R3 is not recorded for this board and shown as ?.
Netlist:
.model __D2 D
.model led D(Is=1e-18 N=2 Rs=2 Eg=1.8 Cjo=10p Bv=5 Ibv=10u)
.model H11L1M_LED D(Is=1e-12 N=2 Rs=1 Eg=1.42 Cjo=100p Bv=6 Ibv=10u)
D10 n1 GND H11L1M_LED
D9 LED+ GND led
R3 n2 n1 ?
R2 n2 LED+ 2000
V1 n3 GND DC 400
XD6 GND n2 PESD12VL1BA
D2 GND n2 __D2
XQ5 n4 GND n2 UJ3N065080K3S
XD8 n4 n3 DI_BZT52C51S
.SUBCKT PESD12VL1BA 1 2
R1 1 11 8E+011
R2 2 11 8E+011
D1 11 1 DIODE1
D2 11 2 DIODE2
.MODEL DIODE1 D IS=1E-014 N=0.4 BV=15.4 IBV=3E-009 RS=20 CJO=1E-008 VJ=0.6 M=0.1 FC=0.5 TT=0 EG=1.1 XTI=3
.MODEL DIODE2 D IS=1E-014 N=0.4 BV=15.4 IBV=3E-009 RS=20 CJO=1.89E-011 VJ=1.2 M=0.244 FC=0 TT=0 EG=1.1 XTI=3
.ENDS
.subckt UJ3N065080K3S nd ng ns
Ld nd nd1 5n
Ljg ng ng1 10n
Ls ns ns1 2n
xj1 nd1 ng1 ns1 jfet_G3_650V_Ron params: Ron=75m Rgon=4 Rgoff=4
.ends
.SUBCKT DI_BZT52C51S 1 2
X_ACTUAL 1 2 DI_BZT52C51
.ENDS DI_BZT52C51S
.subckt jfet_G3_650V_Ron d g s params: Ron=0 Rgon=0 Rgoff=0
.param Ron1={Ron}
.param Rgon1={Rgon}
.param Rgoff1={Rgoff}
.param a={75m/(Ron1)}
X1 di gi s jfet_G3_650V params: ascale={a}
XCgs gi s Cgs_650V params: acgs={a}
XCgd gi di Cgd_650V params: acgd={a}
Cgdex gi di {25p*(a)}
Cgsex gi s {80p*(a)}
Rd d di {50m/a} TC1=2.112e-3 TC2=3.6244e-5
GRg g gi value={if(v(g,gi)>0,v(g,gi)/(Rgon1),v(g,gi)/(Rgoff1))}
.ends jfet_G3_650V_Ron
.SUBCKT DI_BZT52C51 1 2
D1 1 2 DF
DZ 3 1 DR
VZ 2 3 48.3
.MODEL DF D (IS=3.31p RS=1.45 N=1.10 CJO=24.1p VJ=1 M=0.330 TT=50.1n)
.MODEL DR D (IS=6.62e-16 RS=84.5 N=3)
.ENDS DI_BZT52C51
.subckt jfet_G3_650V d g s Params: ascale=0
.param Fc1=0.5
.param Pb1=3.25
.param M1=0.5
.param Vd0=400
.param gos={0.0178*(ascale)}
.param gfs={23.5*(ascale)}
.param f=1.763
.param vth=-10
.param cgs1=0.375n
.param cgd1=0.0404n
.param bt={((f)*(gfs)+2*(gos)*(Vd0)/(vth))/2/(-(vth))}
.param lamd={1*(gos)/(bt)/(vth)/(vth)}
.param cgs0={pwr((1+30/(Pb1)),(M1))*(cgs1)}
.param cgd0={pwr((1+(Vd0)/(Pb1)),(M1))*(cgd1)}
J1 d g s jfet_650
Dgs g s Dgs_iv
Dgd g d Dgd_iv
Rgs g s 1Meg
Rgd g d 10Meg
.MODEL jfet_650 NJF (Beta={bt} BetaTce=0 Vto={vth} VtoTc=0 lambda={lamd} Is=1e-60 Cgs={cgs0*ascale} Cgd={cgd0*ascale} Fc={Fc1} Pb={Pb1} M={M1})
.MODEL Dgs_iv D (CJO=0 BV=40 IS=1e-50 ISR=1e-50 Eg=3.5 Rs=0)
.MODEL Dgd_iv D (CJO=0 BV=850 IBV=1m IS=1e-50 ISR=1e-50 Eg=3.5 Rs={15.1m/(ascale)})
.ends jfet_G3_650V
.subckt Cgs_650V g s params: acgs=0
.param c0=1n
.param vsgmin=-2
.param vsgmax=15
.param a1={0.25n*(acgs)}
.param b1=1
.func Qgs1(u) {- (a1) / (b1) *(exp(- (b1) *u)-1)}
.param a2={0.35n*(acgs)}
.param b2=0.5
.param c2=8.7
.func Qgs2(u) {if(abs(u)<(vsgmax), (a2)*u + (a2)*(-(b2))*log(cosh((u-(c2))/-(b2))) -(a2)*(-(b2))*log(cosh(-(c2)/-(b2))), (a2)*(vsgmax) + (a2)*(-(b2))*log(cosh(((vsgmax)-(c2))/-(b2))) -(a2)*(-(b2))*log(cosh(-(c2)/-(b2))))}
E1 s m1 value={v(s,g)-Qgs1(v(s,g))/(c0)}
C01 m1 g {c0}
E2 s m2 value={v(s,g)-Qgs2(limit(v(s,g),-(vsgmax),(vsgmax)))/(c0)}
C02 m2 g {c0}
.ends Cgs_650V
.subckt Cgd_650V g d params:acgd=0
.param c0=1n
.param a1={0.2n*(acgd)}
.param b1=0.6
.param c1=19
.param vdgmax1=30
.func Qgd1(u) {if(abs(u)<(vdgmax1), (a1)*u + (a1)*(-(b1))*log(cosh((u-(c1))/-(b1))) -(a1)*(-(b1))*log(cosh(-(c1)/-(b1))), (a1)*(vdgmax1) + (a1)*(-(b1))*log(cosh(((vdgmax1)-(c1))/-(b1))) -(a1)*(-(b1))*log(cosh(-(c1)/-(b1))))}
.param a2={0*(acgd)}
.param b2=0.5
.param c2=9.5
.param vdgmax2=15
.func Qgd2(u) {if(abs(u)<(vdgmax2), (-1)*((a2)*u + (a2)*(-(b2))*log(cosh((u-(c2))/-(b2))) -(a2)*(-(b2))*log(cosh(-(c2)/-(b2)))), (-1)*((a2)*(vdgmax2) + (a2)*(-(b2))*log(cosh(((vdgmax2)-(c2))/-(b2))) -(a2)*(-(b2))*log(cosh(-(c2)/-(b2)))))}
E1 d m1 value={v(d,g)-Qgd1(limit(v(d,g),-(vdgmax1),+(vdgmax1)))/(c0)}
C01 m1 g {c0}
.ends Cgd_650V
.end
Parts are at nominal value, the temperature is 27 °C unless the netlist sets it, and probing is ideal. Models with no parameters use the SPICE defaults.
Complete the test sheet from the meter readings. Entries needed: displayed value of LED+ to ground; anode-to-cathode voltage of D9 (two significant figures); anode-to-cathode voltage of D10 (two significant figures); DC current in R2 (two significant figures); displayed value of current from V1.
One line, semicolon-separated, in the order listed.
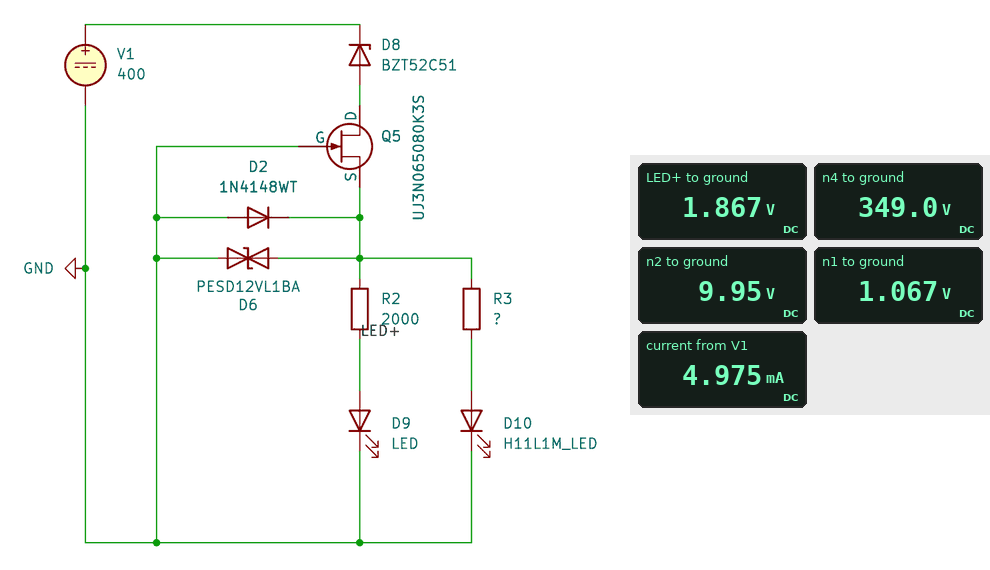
1.867 V; 1.9 V; 1.1 V; 4.0 mA; 4.975 mA
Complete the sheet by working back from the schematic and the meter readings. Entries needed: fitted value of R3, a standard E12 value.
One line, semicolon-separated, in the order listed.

10 kΩ
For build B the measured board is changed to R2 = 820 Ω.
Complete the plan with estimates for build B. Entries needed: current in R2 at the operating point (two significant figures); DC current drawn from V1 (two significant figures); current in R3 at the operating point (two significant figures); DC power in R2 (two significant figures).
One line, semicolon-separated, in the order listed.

9.8 mA; 11 mA; 890 µA; 78 mW
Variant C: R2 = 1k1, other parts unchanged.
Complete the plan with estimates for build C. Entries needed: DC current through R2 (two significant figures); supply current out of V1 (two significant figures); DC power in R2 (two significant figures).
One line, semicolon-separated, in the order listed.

7.3 mA; 8.2 mA; 59 mW
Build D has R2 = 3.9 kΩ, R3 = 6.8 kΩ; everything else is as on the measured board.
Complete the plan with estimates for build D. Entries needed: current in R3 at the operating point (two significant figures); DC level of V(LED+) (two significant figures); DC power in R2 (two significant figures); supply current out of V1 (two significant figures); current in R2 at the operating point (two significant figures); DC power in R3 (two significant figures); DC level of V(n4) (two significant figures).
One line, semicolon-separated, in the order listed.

1.3 mA; 1.8 V; 17 mW; 3.4 mA; 2.1 mA; 12 mW; 350 V
